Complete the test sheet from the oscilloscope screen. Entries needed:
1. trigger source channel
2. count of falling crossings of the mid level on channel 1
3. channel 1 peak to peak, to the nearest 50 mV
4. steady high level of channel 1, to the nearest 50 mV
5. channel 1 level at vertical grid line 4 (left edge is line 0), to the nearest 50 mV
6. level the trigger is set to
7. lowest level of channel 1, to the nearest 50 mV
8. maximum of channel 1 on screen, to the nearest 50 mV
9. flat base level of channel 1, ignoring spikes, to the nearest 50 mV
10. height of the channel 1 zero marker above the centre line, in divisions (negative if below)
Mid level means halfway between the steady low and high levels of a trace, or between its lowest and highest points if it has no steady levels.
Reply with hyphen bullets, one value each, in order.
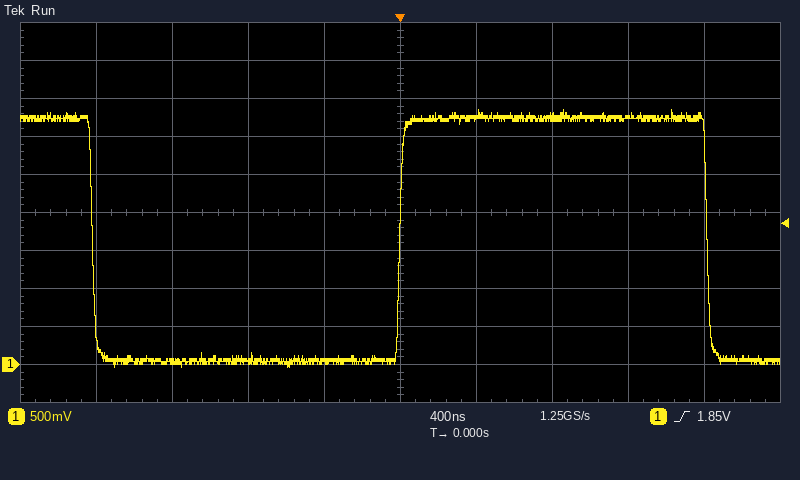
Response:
- channel 1
- 2
- 3.40 V
- 3.25 V
- 50 mV
- 1.85 V
- -50 mV
- 3.35 V
- 50 mV
- -4.0 div
